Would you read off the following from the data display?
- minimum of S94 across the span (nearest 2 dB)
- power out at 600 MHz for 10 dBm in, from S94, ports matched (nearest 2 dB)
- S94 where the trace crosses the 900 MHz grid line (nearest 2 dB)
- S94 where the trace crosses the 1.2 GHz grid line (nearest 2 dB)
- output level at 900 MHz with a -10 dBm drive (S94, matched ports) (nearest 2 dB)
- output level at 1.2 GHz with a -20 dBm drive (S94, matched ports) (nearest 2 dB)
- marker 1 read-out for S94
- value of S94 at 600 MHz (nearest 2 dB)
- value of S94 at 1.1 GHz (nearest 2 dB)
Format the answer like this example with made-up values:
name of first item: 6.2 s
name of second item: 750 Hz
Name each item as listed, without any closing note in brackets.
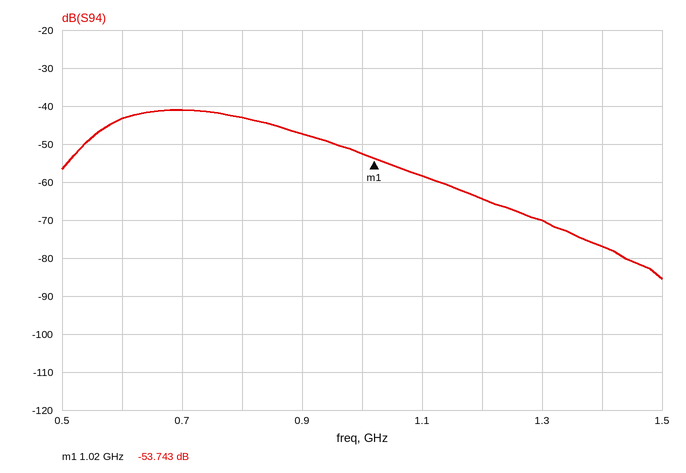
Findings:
minimum of S94 across the span: -86 dB
power out at 600 MHz for 10 dBm in, from S94, ports matched: -34 dBm
S94 where the trace crosses the 900 MHz grid line: -48 dB
S94 where the trace crosses the 1.2 GHz grid line: -64 dB
output level at 900 MHz with a -10 dBm drive (S94, matched ports): -58 dBm
output level at 1.2 GHz with a -20 dBm drive (S94, matched ports): -84 dBm
marker 1 read-out for S94: -53.743 dB
value of S94 at 600 MHz: -44 dB
value of S94 at 1.1 GHz: -58 dB
